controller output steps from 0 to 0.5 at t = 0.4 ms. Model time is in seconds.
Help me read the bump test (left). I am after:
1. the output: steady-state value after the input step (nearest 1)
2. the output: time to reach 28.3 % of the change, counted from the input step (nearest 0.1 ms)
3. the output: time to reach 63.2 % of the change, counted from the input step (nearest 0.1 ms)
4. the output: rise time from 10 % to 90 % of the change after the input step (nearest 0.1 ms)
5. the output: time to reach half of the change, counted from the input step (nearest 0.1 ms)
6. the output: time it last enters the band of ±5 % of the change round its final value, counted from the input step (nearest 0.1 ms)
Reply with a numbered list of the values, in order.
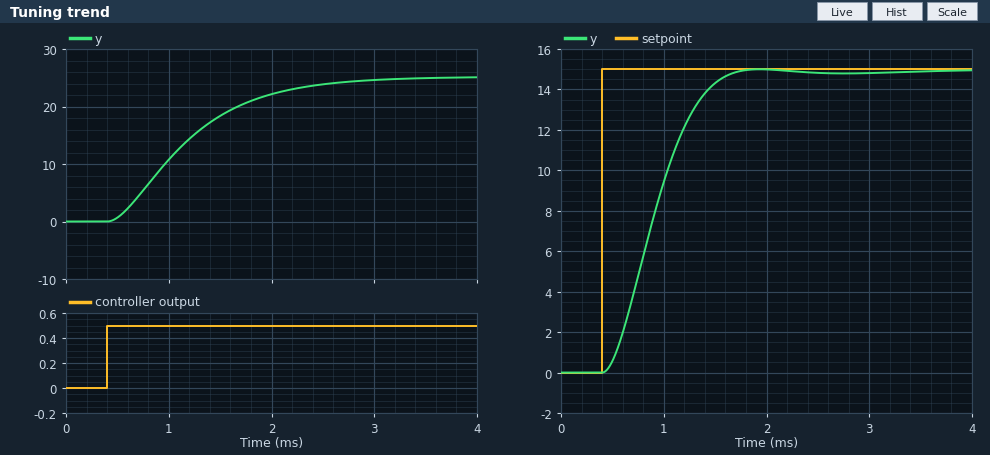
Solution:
1. 25
2. 0.4 ms
3. 0.9 ms
4. 1.5 ms
5. 0.7 ms
6. 2.1 ms
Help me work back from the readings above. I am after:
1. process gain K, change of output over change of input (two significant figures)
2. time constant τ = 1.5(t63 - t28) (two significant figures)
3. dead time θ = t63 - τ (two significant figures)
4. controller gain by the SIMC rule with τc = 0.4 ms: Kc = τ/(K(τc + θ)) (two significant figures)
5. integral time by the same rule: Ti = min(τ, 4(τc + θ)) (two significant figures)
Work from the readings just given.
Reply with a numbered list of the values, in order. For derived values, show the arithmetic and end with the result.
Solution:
1. (25 - 0) / 0.5 = 50
2. 1.5 × (0.9 - 0.4) = 0.75 ms
3. 0.9 - 0.75 = 0.15 ms
4. 0.75 / (50 × (0.4 + 0.15)) = 0.027
5. min(0.75, 4 × (0.4 + 0.15)) = 0.75 ms
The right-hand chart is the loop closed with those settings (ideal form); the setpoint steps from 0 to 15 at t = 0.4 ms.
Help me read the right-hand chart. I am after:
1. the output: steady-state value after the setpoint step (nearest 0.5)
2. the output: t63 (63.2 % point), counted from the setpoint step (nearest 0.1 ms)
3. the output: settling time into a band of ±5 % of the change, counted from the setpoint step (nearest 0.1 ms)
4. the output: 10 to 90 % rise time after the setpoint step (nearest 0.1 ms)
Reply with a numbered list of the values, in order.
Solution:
1. 15.0
2. 0.6 ms
3. 1.1 ms
4. 0.8 ms
